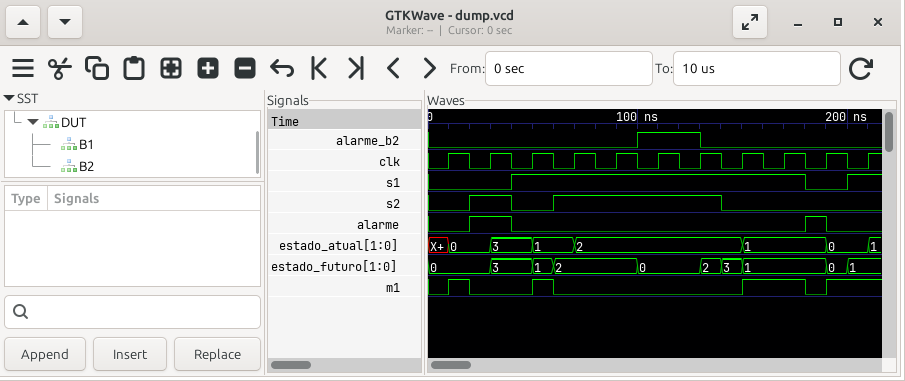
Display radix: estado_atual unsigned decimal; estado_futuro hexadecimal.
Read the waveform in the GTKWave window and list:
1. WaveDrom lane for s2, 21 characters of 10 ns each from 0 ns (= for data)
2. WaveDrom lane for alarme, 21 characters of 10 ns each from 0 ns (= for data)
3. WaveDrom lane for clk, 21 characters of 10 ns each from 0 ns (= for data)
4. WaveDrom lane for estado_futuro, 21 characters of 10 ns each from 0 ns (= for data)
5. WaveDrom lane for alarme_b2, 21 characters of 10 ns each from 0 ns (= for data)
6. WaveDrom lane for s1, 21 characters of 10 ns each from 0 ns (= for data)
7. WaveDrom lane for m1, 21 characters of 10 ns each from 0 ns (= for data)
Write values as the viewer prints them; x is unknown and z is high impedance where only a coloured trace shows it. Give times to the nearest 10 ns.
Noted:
{name: 's2', wave: '0.1.0.1.......0......'}
{name: 'alarme', wave: '0.1.0.............10.'}
{name: 'clk', wave: '010101010101010101010'}
{name: 'estado_futuro', wave: '=..=.==...=..===...==', data: '0 3 1 2 0 2 3 1 0 1'}
{name: 'alarme_b2', wave: '0.........1..0.......'}
{name: 's1', wave: '0...1.............0.1'}
{name: 'm1', wave: '010..10........1..01.'}
